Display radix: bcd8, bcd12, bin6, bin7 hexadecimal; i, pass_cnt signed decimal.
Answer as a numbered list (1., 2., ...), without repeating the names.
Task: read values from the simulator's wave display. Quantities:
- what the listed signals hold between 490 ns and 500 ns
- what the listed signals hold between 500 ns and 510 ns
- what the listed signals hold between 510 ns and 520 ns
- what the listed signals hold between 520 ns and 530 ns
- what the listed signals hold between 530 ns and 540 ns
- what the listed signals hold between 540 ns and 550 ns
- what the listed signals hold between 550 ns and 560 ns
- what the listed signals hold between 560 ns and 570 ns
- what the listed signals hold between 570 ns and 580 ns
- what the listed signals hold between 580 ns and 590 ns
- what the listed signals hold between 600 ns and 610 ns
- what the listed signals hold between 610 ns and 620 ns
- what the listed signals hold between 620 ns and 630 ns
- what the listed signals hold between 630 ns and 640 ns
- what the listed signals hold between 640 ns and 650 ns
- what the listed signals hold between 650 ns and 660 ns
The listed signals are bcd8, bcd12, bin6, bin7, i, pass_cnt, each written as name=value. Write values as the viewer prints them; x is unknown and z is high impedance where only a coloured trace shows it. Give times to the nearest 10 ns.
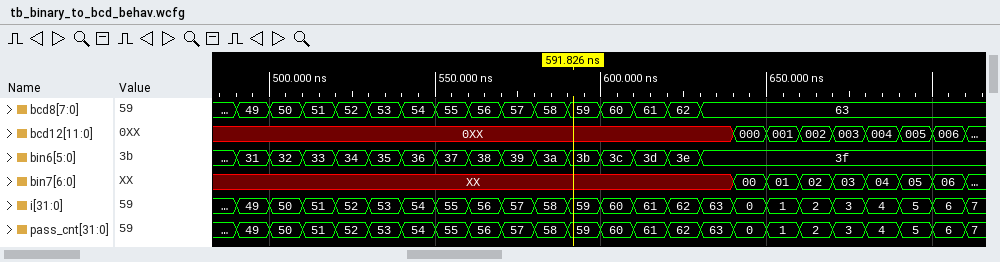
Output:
1. bcd8=49, bcd12=0XX, bin6=31, bin7=XX, i=49, pass_cnt=49
2. bcd8=50, bcd12=0XX, bin6=32, bin7=XX, i=50, pass_cnt=50
3. bcd8=51, bcd12=0XX, bin6=33, bin7=XX, i=51, pass_cnt=51
4. bcd8=52, bcd12=0XX, bin6=34, bin7=XX, i=52, pass_cnt=52
5. bcd8=53, bcd12=0XX, bin6=35, bin7=XX, i=53, pass_cnt=53
6. bcd8=54, bcd12=0XX, bin6=36, bin7=XX, i=54, pass_cnt=54
7. bcd8=55, bcd12=0XX, bin6=37, bin7=XX, i=55, pass_cnt=55
8. bcd8=56, bcd12=0XX, bin6=38, bin7=XX, i=56, pass_cnt=56
9. bcd8=57, bcd12=0XX, bin6=39, bin7=XX, i=57, pass_cnt=57
10. bcd8=58, bcd12=0XX, bin6=3a, bin7=XX, i=58, pass_cnt=58
11. bcd8=60, bcd12=0XX, bin6=3c, bin7=XX, i=60, pass_cnt=60
12. bcd8=61, bcd12=0XX, bin6=3d, bin7=XX, i=61, pass_cnt=61
13. bcd8=62, bcd12=0XX, bin6=3e, bin7=XX, i=62, pass_cnt=62
14. bcd8=63, bcd12=0XX, bin6=3f, bin7=XX, i=63, pass_cnt=63
15. bcd8=63, bcd12=000, bin6=3f, bin7=00, i=0, pass_cnt=0
16. bcd8=63, bcd12=001, bin6=3f, bin7=01, i=1, pass_cnt=1
